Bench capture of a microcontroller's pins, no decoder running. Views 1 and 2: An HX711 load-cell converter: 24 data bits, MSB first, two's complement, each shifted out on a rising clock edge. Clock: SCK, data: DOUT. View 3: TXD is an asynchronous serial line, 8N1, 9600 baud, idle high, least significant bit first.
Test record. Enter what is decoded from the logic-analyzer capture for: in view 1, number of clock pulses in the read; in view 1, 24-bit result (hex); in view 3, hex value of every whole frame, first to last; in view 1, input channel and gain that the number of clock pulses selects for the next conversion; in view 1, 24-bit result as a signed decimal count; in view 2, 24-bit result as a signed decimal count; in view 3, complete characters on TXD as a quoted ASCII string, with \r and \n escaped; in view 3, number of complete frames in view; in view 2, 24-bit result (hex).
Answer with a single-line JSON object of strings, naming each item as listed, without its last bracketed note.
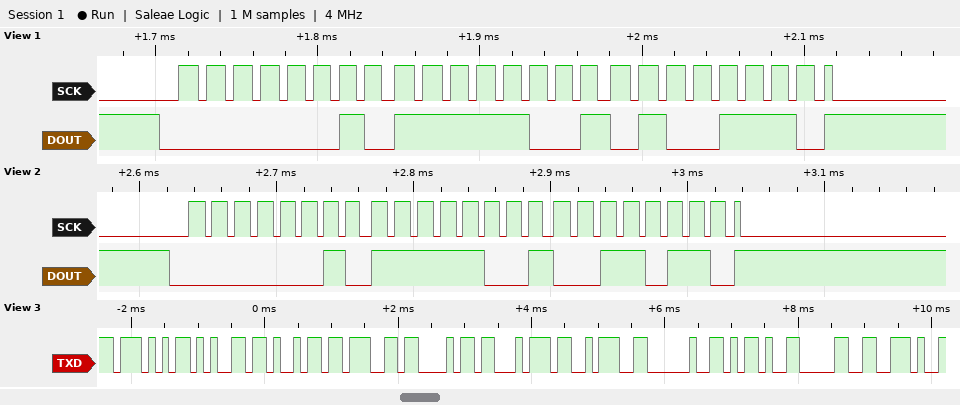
{"in view 1, number of clock pulses in the read": "25", "in view 1, 24-bit result": "0x02F94E", "in view 3, hex value of every whole frame, first to last": "0x57 0x65 0x69 0x67 0x68 0x74 0x3A 0x20 0x2D 0x30 0x2E", "in view 1, input channel and gain that the number of clock pulses selects for the next conversion": "channel A, gain 128", "in view 1, 24-bit result as a signed decimal count": "194894", "in view 2, 24-bit result as a signed decimal count": "194870", "in view 3, complete characters on TXD as a quoted ASCII string, with \\r and \\n escaped": "\"Weight: -0.\"", "in view 3, number of complete frames in view": "11", "in view 2, 24-bit result": "0x02F936"}
